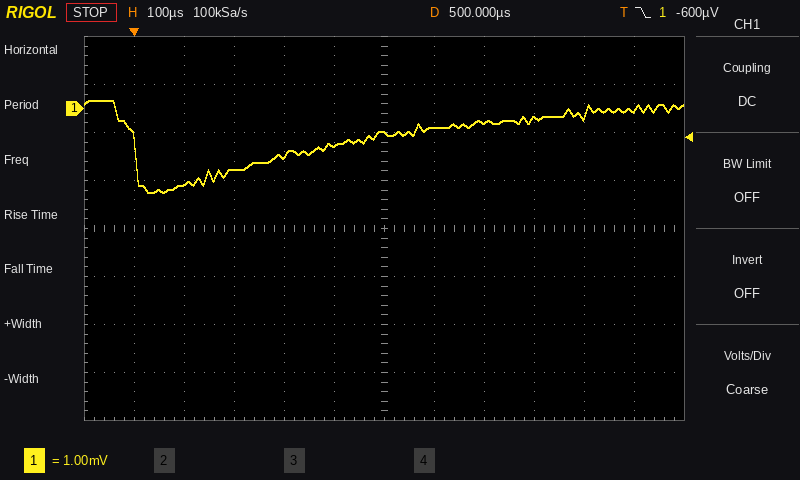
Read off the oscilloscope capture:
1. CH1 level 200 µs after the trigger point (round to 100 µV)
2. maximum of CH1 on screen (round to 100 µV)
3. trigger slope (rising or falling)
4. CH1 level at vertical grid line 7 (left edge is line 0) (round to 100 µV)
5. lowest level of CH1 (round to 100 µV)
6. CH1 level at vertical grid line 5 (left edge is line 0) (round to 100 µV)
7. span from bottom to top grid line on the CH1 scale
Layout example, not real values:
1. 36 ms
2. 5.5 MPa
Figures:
1. -1.3 mV
2. 200 µV
3. falling
4. -400 µV
5. -1.8 mV
6. -800 µV
7. 8 mV
